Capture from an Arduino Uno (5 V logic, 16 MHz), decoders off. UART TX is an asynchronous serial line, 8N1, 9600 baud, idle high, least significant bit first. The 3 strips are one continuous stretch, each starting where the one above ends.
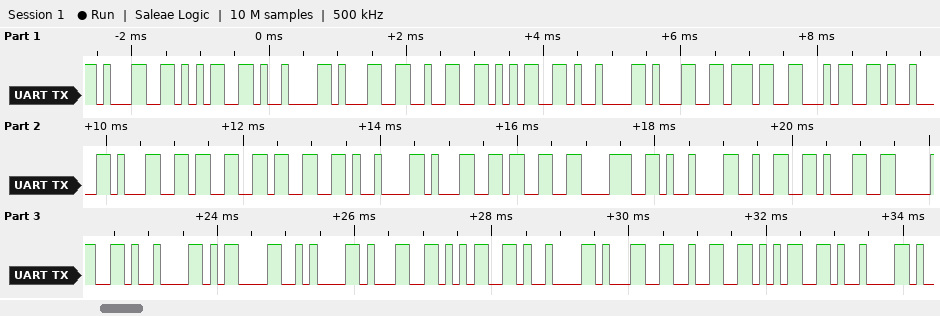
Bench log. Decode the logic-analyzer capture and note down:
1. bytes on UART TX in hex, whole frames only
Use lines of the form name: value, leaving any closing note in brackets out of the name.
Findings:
bytes on UART TX in hex, whole frames only: 31 35 09 31 32 35 09 31 37 34 09 31 33 33 09 31 33 38 09 32 31 30 09 0D 0A 31 35 09 31 32 35 09
